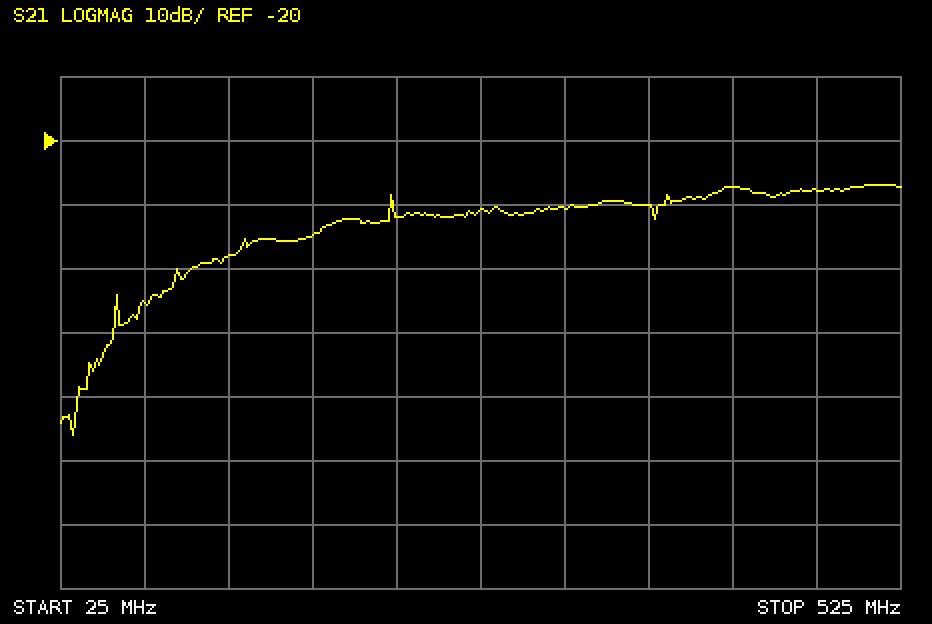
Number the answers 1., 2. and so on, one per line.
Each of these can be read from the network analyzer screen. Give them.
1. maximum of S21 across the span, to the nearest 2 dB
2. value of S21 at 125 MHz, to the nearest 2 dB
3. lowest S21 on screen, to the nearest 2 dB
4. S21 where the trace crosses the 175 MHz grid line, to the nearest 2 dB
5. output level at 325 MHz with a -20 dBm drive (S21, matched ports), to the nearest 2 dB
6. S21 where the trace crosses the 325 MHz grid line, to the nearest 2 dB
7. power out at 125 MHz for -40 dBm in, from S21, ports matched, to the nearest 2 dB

1. -26 dB
2. -38 dB
3. -66 dB
4. -34 dB
5. -50 dBm
6. -30 dB
7. -78 dBm
